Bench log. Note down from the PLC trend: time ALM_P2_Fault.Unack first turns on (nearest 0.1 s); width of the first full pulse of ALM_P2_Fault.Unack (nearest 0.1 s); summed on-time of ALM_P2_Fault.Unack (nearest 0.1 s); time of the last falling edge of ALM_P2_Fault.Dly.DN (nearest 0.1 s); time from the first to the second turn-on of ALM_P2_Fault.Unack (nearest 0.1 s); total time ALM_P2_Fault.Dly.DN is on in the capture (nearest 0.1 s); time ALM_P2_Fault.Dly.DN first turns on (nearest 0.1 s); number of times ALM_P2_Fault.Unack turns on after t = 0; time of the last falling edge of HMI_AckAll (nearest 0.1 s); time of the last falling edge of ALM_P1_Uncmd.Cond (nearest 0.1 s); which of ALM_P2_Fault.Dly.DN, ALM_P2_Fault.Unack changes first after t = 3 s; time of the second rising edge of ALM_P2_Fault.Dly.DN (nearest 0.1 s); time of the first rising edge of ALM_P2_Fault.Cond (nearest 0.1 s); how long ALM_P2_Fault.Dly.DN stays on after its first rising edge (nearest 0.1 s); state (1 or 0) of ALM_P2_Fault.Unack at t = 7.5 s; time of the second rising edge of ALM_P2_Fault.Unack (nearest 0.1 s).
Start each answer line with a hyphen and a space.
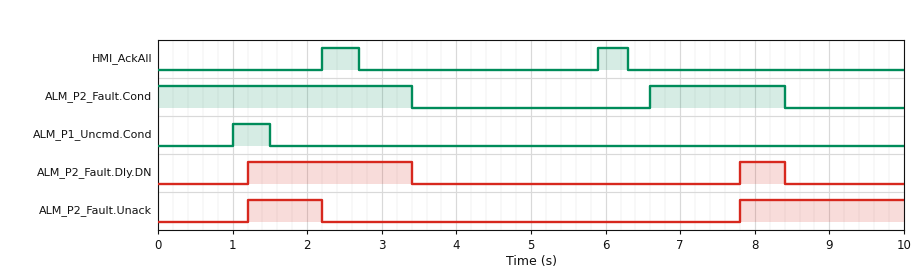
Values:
- 1.2 s
- 1.0 s
- 3.2 s
- 8.4 s
- 6.6 s
- 2.8 s
- 1.2 s
- 2
- 6.3 s
- 1.5 s
- ALM_P2_Fault.Dly.DN
- 7.8 s
- 6.6 s
- 2.2 s
- 0
- 7.8 s
